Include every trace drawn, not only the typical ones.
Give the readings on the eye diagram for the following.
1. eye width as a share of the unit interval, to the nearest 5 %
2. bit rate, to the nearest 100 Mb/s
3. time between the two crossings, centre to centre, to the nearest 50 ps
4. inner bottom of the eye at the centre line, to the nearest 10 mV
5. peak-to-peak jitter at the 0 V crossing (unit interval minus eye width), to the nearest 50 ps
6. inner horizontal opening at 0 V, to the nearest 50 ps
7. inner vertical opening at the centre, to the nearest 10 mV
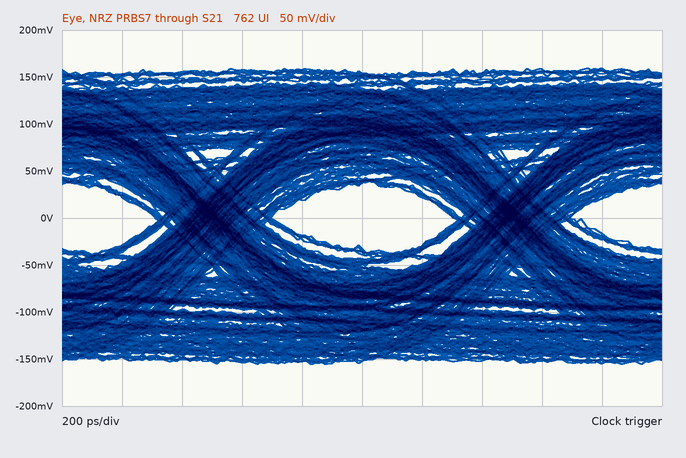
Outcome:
60 %
1.0 Gb/s
1.00 ns
-30 mV
400 ps
600 ps
70 mV
